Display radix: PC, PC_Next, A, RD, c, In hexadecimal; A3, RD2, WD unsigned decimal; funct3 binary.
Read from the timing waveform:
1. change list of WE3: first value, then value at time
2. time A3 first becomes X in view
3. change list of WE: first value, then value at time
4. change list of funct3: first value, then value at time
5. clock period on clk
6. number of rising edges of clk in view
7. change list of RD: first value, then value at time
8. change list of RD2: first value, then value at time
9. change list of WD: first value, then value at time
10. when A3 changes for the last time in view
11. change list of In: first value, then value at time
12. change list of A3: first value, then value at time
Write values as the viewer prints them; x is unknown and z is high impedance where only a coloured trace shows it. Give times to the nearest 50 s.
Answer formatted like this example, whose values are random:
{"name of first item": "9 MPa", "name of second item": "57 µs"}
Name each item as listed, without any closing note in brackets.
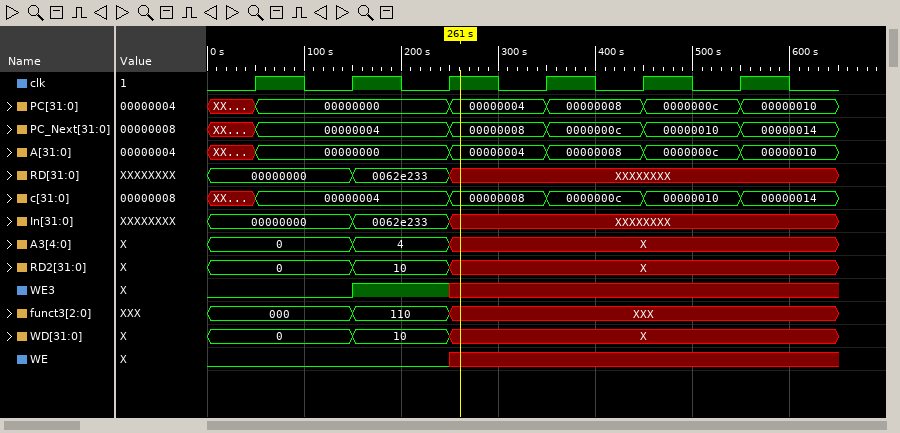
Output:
{"change list of WE3: first value, then value at time": "0, 1 at 150 s, x at 250 s", "time A3 first becomes X in view": "250 s", "change list of WE: first value, then value at time": "0, x at 250 s", "change list of funct3: first value, then value at time": "000, 110 at 150 s, XXX at 250 s", "clock period on clk": "100 s", "number of rising edges of clk in view": "6", "change list of RD: first value, then value at time": "00000000, 0062e233 at 150 s, XXXXXXXX at 250 s", "change list of RD2: first value, then value at time": "0, 10 at 150 s, X at 250 s", "change list of WD: first value, then value at time": "0, 10 at 150 s, X at 250 s", "when A3 changes for the last time in view": "250 s", "change list of In: first value, then value at time": "00000000, 0062e233 at 150 s, XXXXXXXX at 250 s", "change list of A3: first value, then value at time": "0, 4 at 150 s, X at 250 s"}
